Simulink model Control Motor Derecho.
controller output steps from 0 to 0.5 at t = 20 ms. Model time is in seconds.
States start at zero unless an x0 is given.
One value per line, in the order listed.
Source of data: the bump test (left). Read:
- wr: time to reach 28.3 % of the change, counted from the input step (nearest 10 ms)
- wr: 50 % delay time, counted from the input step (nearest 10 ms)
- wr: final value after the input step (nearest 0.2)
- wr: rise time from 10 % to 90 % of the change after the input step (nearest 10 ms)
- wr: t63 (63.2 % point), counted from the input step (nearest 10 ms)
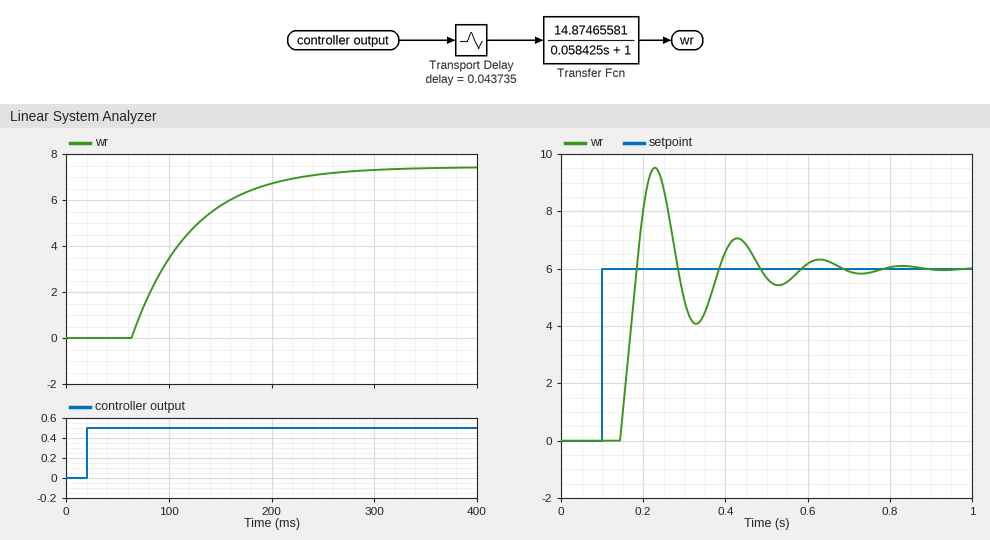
60 ms
80 ms
7.4
130 ms
100 ms
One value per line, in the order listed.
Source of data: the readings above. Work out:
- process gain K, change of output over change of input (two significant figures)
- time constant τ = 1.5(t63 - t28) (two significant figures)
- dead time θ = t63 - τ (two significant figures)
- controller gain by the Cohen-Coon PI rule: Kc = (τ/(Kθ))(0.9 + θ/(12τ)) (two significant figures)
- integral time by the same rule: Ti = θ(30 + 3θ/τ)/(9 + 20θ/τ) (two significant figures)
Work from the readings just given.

15
60 ms
40 ms
0.096
57 ms
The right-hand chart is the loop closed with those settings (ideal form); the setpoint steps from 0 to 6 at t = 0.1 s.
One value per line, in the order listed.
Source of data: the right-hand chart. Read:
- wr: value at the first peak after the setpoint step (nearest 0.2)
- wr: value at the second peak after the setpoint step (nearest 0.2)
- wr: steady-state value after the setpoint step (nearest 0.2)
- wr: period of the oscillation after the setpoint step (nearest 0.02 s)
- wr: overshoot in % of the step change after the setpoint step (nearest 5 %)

9.6
7.0
6.0
0.20 s
60 %
